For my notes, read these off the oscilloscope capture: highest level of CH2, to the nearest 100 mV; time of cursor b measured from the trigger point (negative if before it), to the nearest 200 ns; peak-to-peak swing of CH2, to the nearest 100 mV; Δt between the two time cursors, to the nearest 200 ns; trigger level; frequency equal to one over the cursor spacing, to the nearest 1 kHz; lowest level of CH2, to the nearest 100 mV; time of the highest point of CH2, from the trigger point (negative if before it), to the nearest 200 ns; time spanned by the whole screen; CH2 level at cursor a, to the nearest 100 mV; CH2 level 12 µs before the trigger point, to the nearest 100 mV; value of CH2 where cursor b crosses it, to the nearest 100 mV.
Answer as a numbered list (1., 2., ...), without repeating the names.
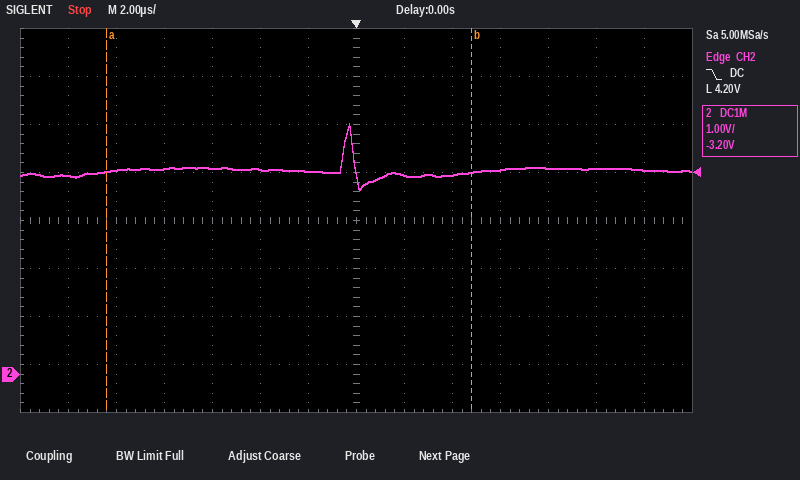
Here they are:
1. 5.2 V
2. +4.8 µs
3. 1.4 V
4. 15.2 µs
5. 4.20 V
6. 66 kHz
7. 3.8 V
8. -200 ns
9. 28 µs
10. 4.2 V
11. 4.1 V
12. 4.2 V
